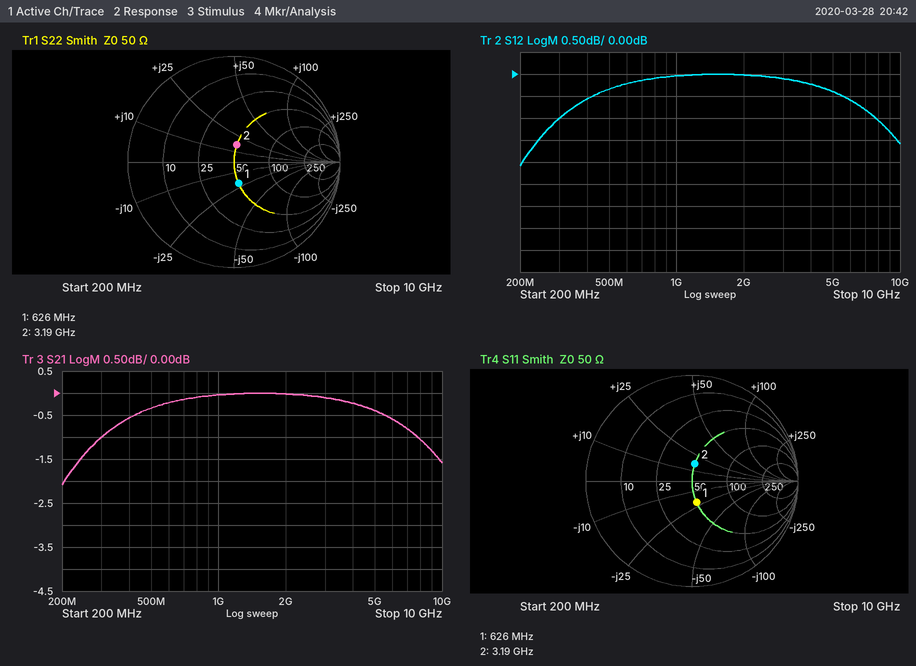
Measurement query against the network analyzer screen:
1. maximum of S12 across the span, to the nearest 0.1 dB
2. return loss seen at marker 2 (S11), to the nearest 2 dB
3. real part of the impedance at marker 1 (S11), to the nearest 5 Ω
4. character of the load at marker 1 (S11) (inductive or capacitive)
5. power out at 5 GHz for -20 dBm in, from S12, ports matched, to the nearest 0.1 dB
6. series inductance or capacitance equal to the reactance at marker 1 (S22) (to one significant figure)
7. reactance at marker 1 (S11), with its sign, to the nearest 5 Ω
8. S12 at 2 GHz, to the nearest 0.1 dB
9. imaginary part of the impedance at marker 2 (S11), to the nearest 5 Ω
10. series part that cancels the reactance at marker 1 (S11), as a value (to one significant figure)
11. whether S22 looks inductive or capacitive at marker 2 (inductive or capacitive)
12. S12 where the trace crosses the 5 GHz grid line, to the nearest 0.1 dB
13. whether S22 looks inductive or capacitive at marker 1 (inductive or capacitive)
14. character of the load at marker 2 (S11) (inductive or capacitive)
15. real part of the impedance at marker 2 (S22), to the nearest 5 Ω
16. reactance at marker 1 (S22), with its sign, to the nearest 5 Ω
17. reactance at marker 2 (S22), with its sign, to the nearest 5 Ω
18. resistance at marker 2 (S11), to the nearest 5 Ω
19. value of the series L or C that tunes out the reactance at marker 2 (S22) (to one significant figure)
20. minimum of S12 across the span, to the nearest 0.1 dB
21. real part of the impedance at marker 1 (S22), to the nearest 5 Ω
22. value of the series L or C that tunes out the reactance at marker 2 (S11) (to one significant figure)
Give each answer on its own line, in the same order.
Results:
0.0 dB
16 dB
50 Ω
capacitive
-20.4 dBm
10 pF
-20 Ω
0.0 dB
+15 Ω
5 nH
inductive
-0.4 dB
capacitive
inductive
50 Ω
-20 Ω
+15 Ω
50 Ω
3 pF
-2.1 dB
50 Ω
3 pF
